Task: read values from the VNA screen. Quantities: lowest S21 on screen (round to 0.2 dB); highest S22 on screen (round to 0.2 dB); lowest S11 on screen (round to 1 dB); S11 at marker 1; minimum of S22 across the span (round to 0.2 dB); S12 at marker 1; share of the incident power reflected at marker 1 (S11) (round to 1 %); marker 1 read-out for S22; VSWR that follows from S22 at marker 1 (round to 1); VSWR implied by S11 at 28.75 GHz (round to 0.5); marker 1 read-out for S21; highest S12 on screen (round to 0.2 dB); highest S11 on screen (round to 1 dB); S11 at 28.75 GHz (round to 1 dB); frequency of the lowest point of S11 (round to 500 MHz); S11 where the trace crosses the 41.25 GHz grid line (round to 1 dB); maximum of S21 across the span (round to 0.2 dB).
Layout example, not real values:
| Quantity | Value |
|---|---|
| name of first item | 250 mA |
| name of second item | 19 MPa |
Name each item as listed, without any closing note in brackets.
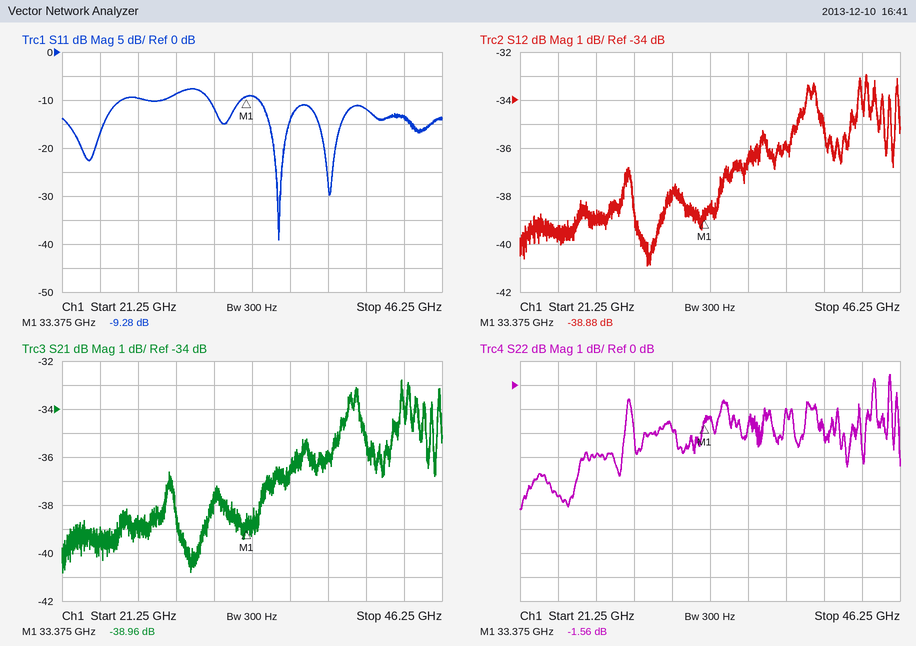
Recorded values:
| Quantity | Value |
|---|---|
| lowest S21 on screen | -40.8 dB |
| highest S22 on screen | 0.4 dB |
| lowest S11 on screen | -39 dB |
| S11 at marker 1 | -9.28 dB |
| minimum of S22 across the span | -5.2 dB |
| S12 at marker 1 | -38.88 dB |
| share of the incident power reflected at marker 1 (S11) | 12 % |
| marker 1 read-out for S22 | -1.56 dB |
| VSWR that follows from S22 at marker 1 | 11 |
| VSWR implied by S11 at 28.75 GHz | 2.0 |
| marker 1 read-out for S21 | -38.96 dB |
| highest S12 on screen | -33.0 dB |
| highest S11 on screen | -8 dB |
| S11 at 28.75 GHz | -9 dB |
| frequency of the lowest point of S11 | 35.5 GHz |
| S11 where the trace crosses the 41.25 GHz grid line | -12 dB |
| maximum of S21 across the span | -32.8 dB |
